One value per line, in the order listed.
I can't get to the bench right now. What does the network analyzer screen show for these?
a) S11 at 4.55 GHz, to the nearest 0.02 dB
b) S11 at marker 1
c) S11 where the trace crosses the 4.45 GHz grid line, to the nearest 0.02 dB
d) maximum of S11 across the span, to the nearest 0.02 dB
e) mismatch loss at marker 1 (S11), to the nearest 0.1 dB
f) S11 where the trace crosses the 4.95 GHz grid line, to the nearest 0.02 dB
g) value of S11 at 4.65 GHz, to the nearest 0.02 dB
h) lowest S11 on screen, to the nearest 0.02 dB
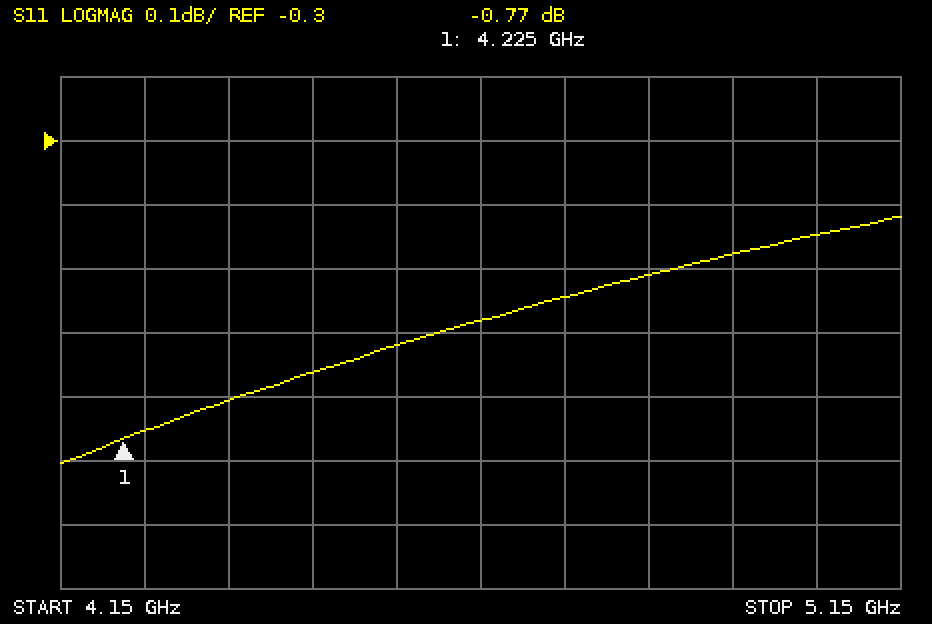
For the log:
-0.62 dB
-0.77 dB
-0.66 dB
-0.42 dB
7.9 dB
-0.48 dB
-0.58 dB
-0.80 dB
